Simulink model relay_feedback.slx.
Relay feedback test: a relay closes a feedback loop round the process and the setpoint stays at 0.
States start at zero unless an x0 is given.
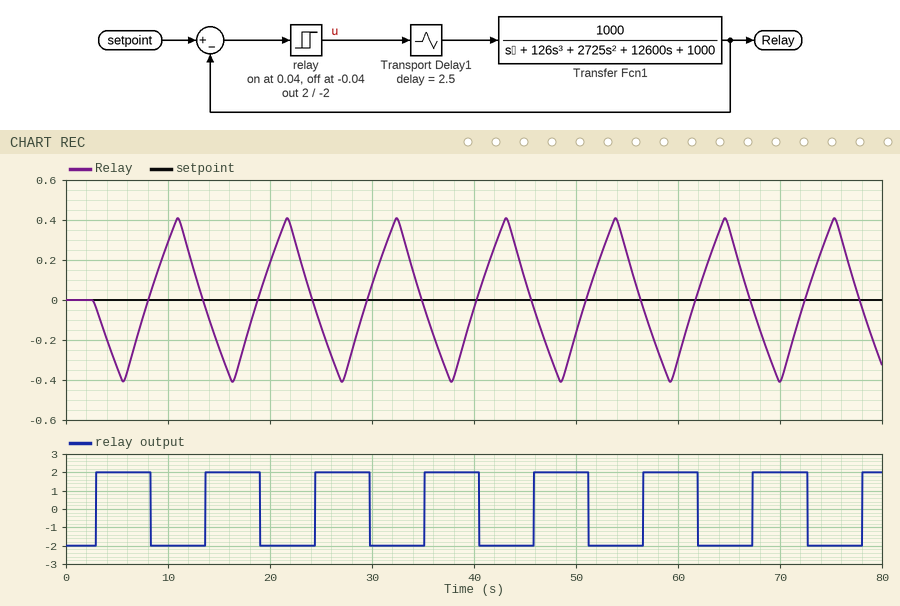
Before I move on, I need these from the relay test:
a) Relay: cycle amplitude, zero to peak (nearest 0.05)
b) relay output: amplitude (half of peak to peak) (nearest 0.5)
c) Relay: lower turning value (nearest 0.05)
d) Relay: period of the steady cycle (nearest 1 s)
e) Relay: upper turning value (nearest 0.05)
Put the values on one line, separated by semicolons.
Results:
0.40; 2.0; -0.40; 11 s; 0.40
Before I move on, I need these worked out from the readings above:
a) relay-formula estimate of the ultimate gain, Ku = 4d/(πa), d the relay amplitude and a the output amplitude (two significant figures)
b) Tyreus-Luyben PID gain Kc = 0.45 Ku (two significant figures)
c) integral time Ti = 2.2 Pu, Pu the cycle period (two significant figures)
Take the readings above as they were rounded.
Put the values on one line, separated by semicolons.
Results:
6.4; 2.9; 24 s
